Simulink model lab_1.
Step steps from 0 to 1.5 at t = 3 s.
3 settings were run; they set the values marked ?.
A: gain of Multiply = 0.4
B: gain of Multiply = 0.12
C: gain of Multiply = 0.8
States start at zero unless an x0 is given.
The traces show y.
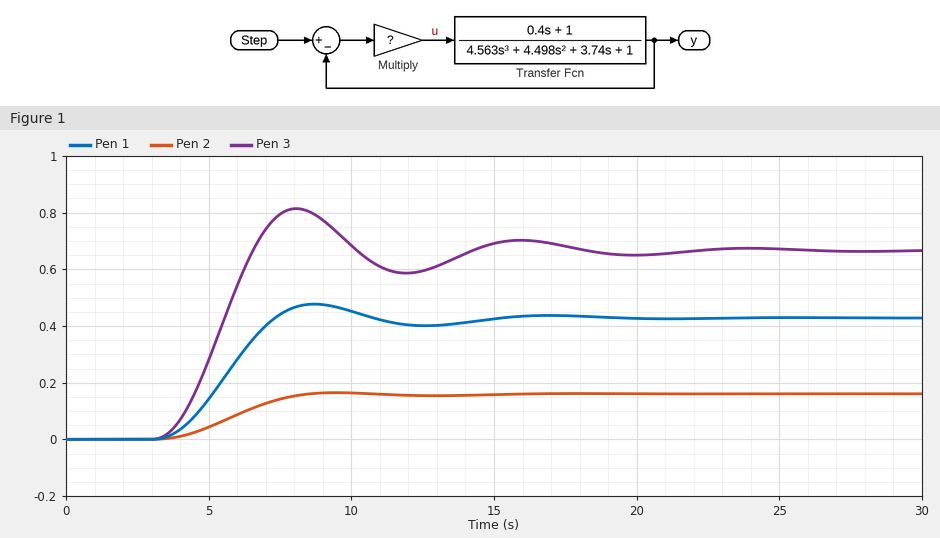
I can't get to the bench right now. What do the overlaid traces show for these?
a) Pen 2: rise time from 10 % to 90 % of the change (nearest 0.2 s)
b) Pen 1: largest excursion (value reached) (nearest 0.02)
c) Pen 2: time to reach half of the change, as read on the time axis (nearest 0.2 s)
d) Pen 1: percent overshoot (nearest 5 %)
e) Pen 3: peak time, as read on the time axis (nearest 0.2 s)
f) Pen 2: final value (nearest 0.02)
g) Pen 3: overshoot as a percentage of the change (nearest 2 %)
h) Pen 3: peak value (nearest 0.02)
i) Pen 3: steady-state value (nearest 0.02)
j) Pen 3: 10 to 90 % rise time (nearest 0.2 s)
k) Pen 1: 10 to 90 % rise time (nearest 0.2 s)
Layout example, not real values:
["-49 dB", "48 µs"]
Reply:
["3.4 s", "0.48", "5.8 s", "10 %", "8.0 s", "0.16", "22 %", "0.82", "0.66", "2.2 s", "2.8 s"]
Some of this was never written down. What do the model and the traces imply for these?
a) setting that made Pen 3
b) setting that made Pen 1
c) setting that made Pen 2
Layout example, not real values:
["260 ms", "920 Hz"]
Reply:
["C", "A", "B"]
